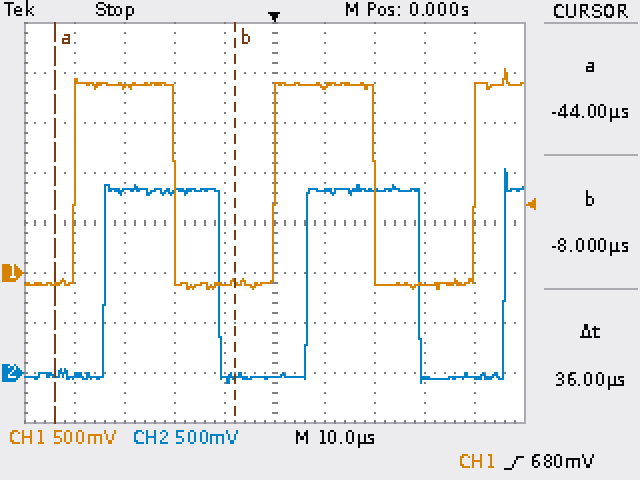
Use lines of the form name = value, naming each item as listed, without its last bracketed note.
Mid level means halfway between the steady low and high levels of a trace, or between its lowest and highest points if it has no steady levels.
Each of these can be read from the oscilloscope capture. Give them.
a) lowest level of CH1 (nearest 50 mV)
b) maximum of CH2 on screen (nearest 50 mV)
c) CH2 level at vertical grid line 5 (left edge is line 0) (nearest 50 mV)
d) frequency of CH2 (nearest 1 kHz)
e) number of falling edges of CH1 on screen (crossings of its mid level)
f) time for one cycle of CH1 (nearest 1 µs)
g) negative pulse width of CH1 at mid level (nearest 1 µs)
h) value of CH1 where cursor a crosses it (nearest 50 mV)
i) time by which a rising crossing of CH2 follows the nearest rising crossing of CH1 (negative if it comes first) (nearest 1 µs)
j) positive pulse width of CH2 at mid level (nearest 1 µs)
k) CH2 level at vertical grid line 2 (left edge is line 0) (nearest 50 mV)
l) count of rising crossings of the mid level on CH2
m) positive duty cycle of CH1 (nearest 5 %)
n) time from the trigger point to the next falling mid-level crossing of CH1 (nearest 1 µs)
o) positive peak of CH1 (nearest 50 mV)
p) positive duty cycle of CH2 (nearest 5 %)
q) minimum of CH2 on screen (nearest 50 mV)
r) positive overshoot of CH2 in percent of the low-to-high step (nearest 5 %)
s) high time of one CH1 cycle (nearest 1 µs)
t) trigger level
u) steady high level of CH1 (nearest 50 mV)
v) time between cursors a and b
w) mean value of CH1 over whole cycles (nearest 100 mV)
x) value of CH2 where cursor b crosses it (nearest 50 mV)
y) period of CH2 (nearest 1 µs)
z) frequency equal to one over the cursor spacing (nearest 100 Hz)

lowest level of CH1 = -150 mV
maximum of CH2 on screen = 2.05 V
CH2 level at vertical grid line 5 (left edge is line 0) = -50 mV
frequency of CH2 = 25 kHz
number of falling edges of CH1 on screen = 2
time for one cycle of CH1 = 40 µs
negative pulse width of CH1 at mid level = 20 µs
value of CH1 where cursor a crosses it = -100 mV
time by which a rising crossing of CH2 follows the nearest rising crossing of CH1 (negative if it comes first) = +6 µs
positive pulse width of CH2 at mid level = 23 µs
CH2 level at vertical grid line 2 (left edge is line 0) = 1.80 V
count of rising crossings of the mid level on CH2 = 3
positive duty cycle of CH1 = 50 %
time from the trigger point to the next falling mid-level crossing of CH1 = 20 µs
positive peak of CH1 = 2.05 V
positive duty cycle of CH2 = 55 %
minimum of CH2 on screen = -100 mV
positive overshoot of CH2 in percent of the low-to-high step = 10 %
high time of one CH1 cycle = 20 µs
trigger level = 680 mV
steady high level of CH1 = 1.90 V
time between cursors a and b = 36 µs
mean value of CH1 over whole cycles = 900 mV
value of CH2 where cursor b crosses it = -50 mV
period of CH2 = 40 µs
frequency equal to one over the cursor spacing = 27.8 kHz
